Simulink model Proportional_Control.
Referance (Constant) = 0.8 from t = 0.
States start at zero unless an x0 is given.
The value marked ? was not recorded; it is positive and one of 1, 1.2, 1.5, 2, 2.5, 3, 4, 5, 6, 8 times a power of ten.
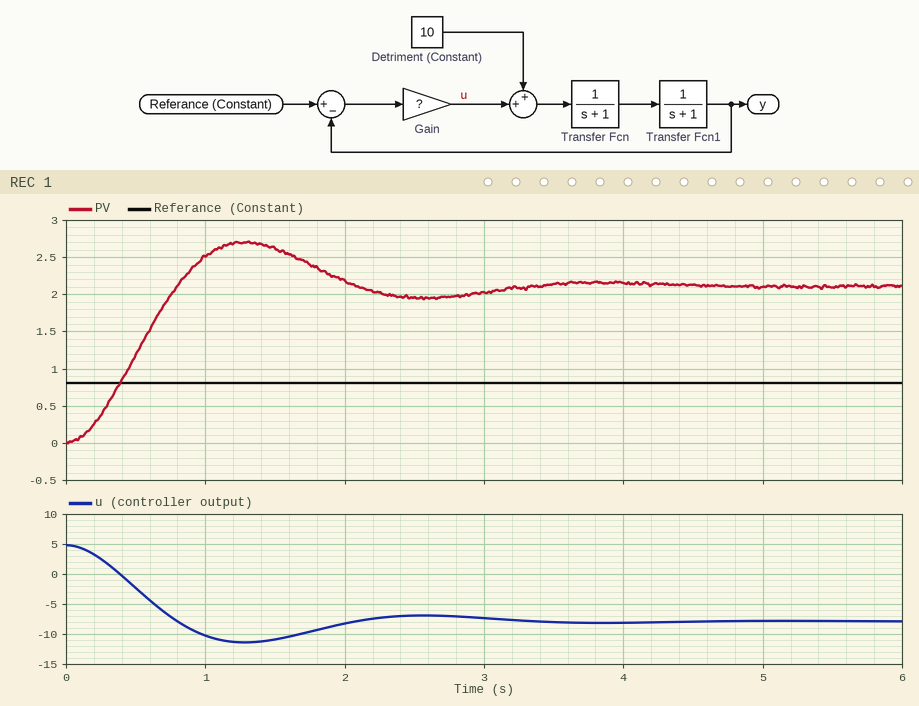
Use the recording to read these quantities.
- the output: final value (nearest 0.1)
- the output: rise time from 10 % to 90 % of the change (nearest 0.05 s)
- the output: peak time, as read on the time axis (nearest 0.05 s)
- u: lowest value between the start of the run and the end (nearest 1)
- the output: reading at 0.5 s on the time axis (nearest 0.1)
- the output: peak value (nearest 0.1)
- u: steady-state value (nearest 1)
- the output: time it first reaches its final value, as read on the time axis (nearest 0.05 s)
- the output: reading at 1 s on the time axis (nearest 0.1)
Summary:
2.1
0.55 s
1.30 s
-11
1.2
2.7
-8
0.80 s
2.5
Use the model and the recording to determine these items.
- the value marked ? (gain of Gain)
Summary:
6
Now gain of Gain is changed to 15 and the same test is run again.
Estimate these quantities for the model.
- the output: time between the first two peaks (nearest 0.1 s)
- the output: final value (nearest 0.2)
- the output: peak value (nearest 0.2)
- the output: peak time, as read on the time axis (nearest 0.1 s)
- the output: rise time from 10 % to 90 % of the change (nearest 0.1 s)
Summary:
1.6 s
1.4
2.0
0.8 s
0.3 s
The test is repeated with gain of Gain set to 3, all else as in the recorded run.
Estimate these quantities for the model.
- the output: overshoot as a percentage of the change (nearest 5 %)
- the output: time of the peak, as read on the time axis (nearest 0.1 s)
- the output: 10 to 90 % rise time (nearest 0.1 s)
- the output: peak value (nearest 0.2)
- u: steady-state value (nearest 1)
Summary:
15 %
1.8 s
0.8 s
3.6
-7
